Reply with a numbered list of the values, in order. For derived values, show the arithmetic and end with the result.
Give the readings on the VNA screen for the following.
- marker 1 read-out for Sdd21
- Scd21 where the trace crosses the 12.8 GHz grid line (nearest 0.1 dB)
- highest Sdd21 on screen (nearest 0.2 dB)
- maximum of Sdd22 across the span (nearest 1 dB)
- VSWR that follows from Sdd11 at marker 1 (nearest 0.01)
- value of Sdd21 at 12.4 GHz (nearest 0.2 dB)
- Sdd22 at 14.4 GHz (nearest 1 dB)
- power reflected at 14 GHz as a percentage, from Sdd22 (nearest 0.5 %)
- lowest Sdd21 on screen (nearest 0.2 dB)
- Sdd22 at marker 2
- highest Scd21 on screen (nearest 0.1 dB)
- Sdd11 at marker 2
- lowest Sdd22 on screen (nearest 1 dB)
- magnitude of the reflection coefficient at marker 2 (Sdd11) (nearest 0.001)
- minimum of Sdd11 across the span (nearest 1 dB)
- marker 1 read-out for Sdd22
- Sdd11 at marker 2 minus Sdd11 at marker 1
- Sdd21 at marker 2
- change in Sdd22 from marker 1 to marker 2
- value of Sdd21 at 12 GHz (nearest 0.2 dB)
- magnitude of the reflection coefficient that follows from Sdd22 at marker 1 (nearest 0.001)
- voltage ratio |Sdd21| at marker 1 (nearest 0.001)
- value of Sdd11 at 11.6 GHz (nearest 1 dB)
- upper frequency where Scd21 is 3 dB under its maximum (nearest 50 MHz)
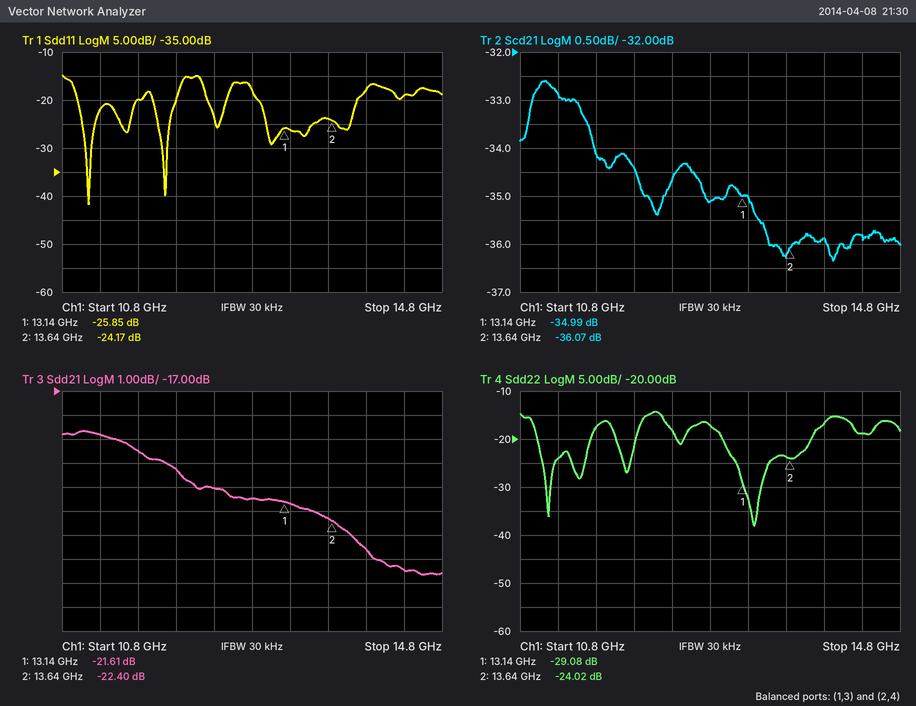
1. -21.61 dB
2. -35.1 dB
3. -18.6 dB
4. -14 dB
5. (1 + 0.0510)/(1 − 0.0510) ≈ 1.11
6. -21.0 dB
7. -19 dB
8. 10^(-17/10) ≈ 2.0 %
9. -24.6 dB
10. -24.02 dB
11. -32.6 dB
12. -24.17 dB
13. -38 dB
14. 10^(-24.17/20) ≈ 0.062
15. -42 dB
16. -29.08 dB
17. -24.17 − (-25.85) = 1.68 dB
18. -22.40 dB
19. -24.02 − (-29.08) = 5.06 dB
20. -20.2 dB
21. 10^(-29.08/20) ≈ 0.035
22. 10^(-21.61/20) ≈ 0.083
23. -20 dB
24. 13.35 GHz
